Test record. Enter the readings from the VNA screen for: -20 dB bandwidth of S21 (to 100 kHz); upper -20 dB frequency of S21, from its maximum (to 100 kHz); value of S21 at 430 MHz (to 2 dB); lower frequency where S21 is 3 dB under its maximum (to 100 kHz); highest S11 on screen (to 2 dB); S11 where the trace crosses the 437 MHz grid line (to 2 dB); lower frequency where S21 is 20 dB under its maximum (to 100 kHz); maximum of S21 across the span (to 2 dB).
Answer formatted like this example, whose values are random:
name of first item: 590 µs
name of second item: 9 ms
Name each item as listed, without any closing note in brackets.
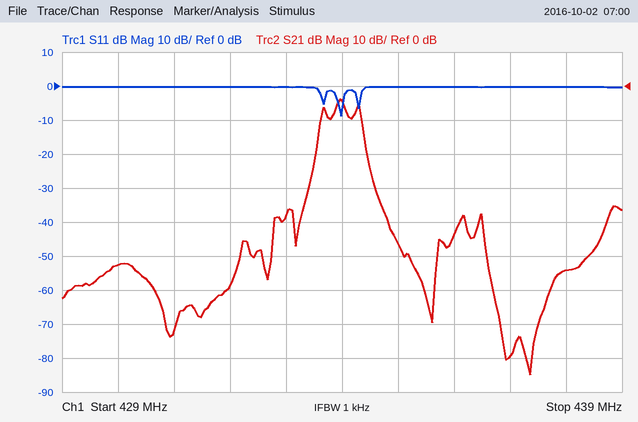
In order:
-20 dB bandwidth of S21: 1.0 MHz
upper -20 dB frequency of S21, from its maximum: 434.5 MHz
value of S21 at 430 MHz: -52 dB
lower frequency where S21 is 3 dB under its maximum: 433.9 MHz
highest S11 on screen: 0 dB
S11 where the trace crosses the 437 MHz grid line: 0 dB
lower frequency where S21 is 20 dB under its maximum: 433.5 MHz
maximum of S21 across the span: -4 dB
